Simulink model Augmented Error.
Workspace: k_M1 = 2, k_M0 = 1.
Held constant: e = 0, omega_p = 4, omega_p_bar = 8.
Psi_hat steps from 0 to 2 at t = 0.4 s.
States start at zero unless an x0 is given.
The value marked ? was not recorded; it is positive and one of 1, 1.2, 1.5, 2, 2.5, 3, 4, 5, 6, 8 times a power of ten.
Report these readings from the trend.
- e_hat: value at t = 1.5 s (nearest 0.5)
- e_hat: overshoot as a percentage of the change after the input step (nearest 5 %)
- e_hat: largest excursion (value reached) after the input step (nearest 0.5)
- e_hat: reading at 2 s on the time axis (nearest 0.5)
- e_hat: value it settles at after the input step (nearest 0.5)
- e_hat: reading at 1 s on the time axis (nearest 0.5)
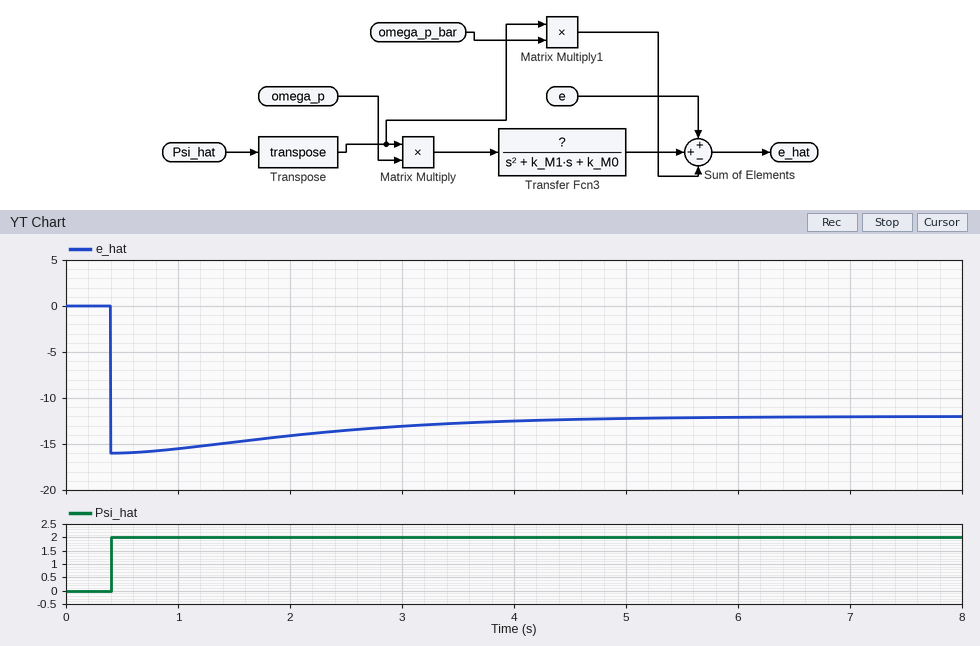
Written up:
-15.0
35 %
-16.0
-14.0
-12.0
-15.5
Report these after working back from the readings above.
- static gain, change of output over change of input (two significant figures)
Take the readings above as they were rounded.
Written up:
-6.0
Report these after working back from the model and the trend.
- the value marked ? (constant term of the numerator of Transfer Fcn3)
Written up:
0.5
